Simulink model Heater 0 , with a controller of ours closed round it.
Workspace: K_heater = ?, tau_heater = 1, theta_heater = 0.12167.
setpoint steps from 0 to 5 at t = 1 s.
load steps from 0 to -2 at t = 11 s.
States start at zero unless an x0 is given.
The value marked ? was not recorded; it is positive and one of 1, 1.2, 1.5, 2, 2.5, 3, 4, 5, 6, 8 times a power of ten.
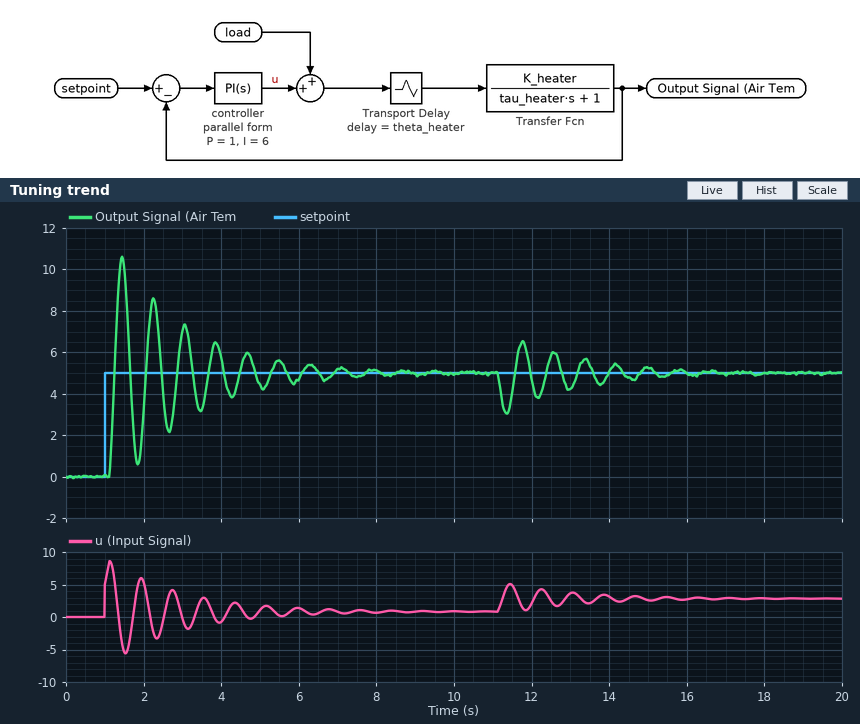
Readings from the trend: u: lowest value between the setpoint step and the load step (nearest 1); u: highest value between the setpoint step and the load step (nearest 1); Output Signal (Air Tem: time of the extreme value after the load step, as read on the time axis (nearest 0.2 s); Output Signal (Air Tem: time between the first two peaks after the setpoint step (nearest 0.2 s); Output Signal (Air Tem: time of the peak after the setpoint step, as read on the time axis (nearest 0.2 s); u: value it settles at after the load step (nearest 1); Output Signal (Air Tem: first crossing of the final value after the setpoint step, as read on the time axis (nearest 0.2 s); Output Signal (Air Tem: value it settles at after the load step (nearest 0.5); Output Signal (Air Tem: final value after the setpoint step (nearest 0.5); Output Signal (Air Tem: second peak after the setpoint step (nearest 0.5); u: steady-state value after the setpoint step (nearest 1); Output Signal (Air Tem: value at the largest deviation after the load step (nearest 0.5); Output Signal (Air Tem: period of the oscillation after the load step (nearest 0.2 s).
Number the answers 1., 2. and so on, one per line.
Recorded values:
1. -6
2. 9
3. 11.4 s
4. 0.8 s
5. 1.4 s
6. 3
7. 1.2 s
8. 5.0
9. 5.0
10. 8.5
11. 1
12. 3.0
13. 0.8 s
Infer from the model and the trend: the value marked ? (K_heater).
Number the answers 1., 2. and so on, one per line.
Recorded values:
1. 6
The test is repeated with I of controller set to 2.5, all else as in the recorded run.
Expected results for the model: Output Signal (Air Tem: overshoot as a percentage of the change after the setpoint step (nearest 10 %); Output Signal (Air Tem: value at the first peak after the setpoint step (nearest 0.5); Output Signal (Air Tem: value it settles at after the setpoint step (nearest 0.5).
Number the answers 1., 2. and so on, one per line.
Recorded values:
1. 50 %
2. 7.5
3. 5.0
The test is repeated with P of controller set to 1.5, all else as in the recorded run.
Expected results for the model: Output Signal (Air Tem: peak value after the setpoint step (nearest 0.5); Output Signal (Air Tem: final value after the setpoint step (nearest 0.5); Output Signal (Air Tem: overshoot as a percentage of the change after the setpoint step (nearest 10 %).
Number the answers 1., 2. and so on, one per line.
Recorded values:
1. 11.0
2. 5.0
3. 120 %
